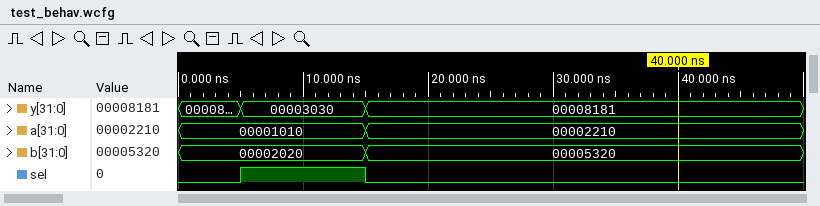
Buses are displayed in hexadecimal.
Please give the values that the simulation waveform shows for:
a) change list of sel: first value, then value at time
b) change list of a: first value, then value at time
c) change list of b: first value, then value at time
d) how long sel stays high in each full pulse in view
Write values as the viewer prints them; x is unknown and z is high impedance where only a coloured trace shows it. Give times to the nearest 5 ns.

0, 1 at 5 ns, 0 at 15 ns
00001010, 00002210 at 15 ns
00002020, 00005320 at 15 ns
10 ns
